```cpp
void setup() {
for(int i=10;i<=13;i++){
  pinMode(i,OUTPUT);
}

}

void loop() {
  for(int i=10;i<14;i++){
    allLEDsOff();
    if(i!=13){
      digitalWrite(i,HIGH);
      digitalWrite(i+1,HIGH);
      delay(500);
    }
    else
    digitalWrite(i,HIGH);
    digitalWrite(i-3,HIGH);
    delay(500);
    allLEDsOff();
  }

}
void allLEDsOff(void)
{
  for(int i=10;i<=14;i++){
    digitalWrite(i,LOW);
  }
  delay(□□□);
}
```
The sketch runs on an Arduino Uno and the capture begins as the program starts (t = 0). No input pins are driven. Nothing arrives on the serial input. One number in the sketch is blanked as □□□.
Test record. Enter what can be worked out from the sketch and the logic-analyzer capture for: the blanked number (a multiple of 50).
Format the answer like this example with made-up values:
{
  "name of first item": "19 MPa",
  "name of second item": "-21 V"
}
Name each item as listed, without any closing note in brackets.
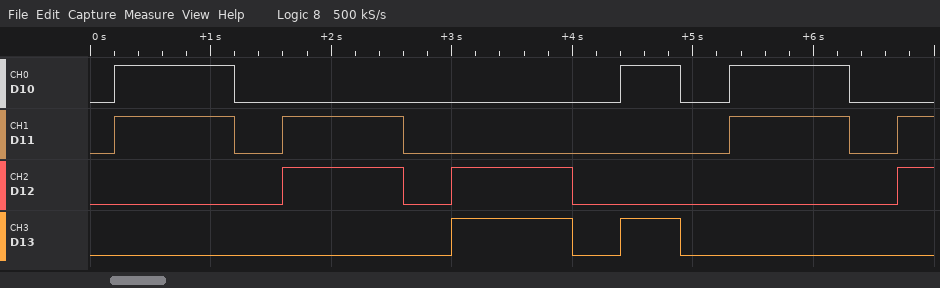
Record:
{
  "the blanked number": "200"
}
